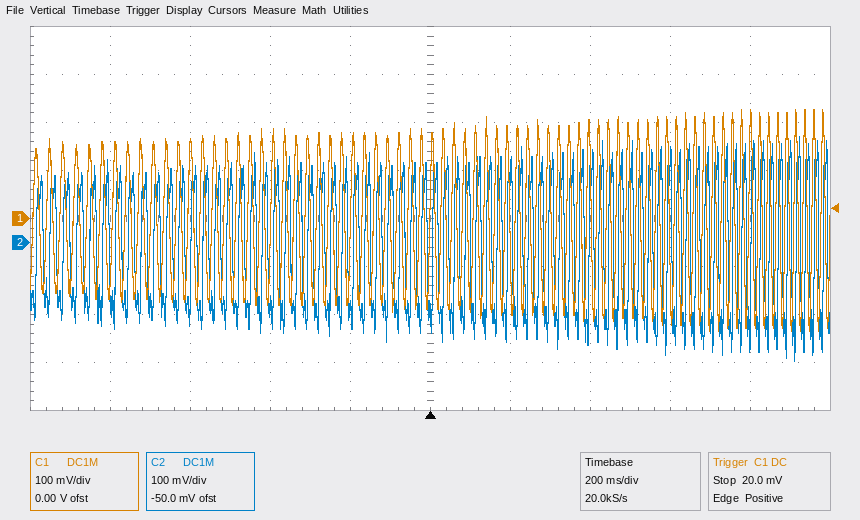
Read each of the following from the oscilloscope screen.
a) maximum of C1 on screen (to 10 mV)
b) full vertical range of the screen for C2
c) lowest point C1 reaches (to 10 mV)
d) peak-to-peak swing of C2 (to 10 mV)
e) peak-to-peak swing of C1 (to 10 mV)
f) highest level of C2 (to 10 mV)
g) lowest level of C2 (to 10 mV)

230 mV
800 mV
-230 mV
470 mV
460 mV
220 mV
-250 mV
